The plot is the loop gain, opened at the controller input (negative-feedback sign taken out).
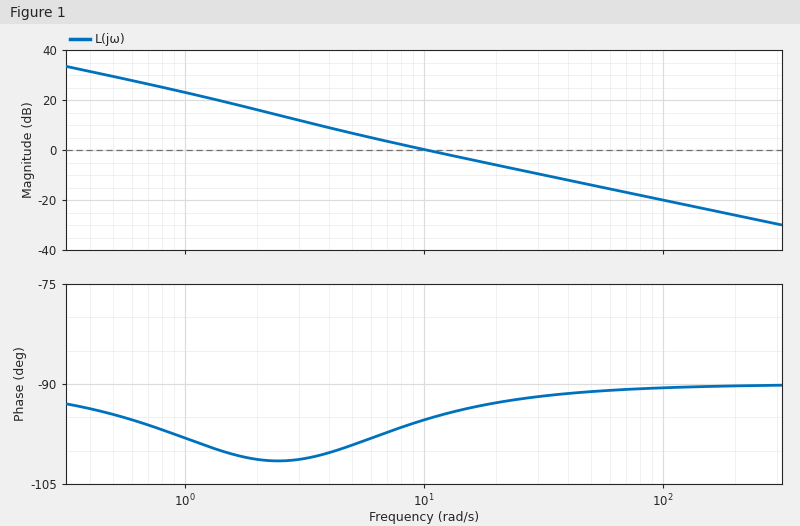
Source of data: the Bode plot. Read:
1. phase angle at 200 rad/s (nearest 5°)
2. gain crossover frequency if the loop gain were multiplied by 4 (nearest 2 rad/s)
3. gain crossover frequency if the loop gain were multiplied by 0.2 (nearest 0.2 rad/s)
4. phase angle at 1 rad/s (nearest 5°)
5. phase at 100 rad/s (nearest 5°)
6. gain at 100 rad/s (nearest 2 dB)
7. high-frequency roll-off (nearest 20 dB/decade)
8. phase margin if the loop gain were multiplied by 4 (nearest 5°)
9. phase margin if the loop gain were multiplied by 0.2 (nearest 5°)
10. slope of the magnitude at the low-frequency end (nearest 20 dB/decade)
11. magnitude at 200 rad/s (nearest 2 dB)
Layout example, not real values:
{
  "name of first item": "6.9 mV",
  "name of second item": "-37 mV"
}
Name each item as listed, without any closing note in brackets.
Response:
{
  "phase angle at 200 rad/s": "-90°",
  "gain crossover frequency if the loop gain were multiplied by 4": "40 rad/s",
  "gain crossover frequency if the loop gain were multiplied by 0.2": "2.4 rad/s",
  "phase angle at 1 rad/s": "-100°",
  "phase at 100 rad/s": "-90°",
  "gain at 100 rad/s": "-20 dB",
  "high-frequency roll-off": "-20 dB/decade",
  "phase margin if the loop gain were multiplied by 4": "90°",
  "phase margin if the loop gain were multiplied by 0.2": "80°",
  "slope of the magnitude at the low-frequency end": "-20 dB/decade",
  "magnitude at 200 rad/s": "-26 dB"
}
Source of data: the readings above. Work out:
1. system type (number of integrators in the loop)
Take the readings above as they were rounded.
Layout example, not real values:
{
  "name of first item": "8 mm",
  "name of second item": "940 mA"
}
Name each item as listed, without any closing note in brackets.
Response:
{
  "system type": "1"
}
